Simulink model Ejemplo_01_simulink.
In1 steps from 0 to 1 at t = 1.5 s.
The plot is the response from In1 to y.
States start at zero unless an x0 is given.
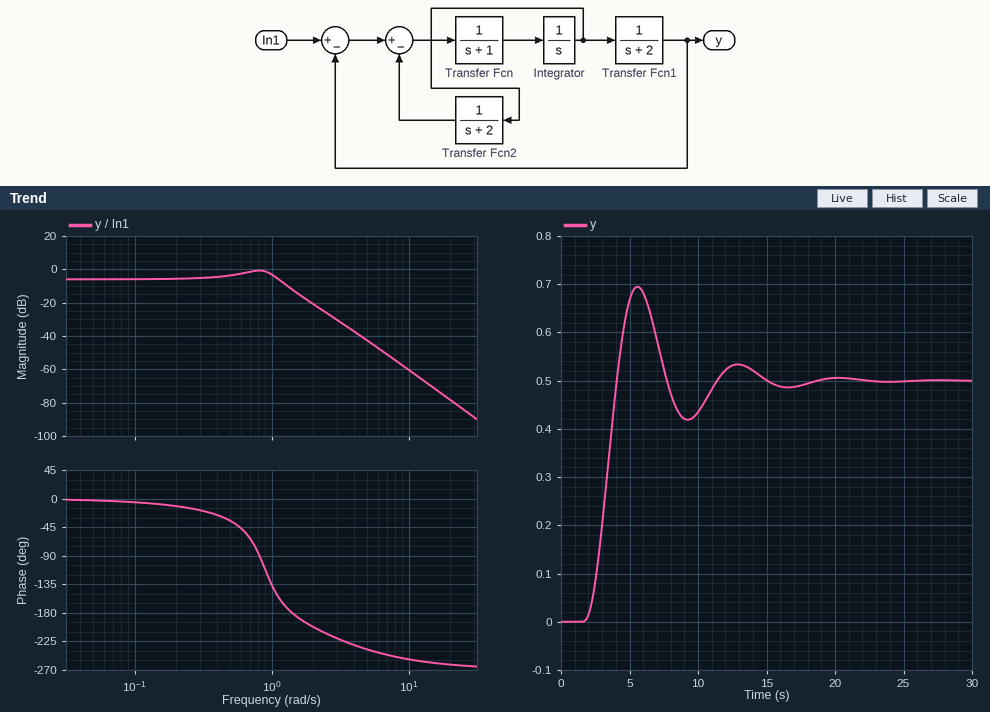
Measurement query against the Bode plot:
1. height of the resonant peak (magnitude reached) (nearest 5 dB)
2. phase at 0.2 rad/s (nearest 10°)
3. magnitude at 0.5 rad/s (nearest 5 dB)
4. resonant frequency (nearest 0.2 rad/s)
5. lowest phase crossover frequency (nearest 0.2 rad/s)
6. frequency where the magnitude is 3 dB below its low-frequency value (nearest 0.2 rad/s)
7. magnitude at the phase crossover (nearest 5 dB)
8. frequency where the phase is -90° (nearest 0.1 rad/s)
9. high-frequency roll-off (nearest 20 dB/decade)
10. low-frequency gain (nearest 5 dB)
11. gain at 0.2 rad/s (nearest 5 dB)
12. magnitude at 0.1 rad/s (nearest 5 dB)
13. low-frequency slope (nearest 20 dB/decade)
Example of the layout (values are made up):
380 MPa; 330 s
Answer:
0 dB; -10°; -5 dB; 0.8 rad/s; 1.4 rad/s; 1.2 rad/s; -10 dB; 0.8 rad/s; -60 dB/decade; -5 dB; -5 dB; -5 dB; 0 dB/decade
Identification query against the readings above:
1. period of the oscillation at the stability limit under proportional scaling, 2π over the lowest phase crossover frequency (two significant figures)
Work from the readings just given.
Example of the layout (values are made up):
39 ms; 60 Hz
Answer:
4.5 s
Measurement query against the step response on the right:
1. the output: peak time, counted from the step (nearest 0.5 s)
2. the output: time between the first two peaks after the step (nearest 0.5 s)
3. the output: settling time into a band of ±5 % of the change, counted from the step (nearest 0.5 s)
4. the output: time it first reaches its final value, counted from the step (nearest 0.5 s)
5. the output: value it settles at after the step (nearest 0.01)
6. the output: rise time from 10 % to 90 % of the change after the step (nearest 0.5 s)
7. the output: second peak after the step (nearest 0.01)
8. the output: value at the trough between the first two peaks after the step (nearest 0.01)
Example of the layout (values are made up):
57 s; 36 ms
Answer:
4.0 s; 7.5 s; 12.5 s; 2.5 s; 0.50; 1.5 s; 0.53; 0.42
